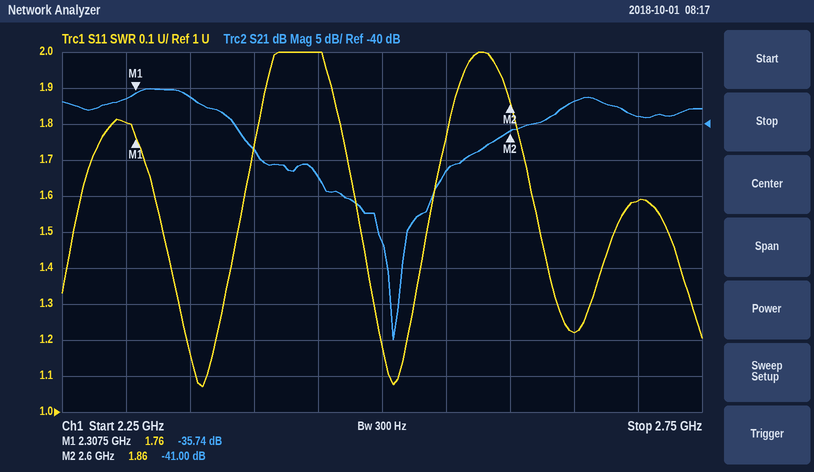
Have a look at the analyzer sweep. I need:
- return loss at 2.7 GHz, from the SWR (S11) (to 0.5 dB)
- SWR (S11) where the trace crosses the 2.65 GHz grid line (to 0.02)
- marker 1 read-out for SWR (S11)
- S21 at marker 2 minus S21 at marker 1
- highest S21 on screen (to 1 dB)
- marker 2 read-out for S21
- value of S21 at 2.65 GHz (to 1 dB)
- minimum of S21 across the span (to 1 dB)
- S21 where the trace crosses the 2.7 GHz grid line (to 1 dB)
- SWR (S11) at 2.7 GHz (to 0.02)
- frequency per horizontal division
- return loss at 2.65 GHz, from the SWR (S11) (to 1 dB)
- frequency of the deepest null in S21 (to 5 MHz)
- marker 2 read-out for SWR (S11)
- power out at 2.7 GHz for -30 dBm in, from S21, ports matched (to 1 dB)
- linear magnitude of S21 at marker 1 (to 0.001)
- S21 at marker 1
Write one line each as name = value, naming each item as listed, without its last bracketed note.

return loss at 2.7 GHz, from the SWR (S11) = 13.0 dB
SWR (S11) where the trace crosses the 2.65 GHz grid line = 1.22
marker 1 read-out for SWR = 1.76
S21 at marker 2 minus S21 at marker 1 = -5.26 dB
highest S21 on screen = -35 dB
marker 2 read-out for S21 = -41.00 dB
value of S21 at 2.65 GHz = -37 dB
minimum of S21 across the span = -70 dB
S21 where the trace crosses the 2.7 GHz grid line = -39 dB
SWR (S11) at 2.7 GHz = 1.58
frequency per horizontal division = 50 MHz
return loss at 2.65 GHz, from the SWR (S11) = 20 dB
frequency of the deepest null in S21 = 2.510 GHz
marker 2 read-out for SWR = 1.86
power out at 2.7 GHz for -30 dBm in, from S21, ports matched = -69 dBm
linear magnitude of S21 at marker 1 = 0.016
S21 at marker 1 = -35.74 dB
